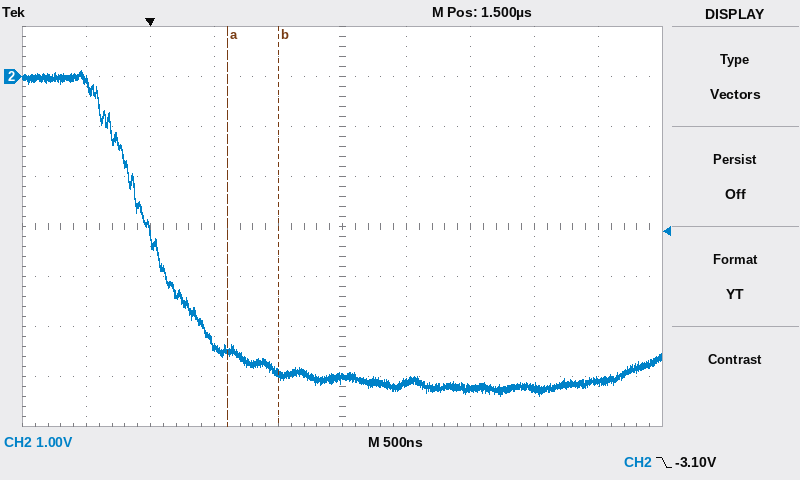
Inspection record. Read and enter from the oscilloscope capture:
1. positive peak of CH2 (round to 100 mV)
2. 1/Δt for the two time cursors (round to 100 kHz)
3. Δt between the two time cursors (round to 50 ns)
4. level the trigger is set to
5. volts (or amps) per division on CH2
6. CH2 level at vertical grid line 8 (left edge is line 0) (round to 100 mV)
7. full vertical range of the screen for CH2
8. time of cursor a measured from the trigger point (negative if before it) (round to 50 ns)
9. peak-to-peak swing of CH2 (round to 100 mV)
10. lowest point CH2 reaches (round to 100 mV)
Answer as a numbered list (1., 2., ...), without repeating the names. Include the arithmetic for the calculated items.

1. 100 mV
2. 1 / 400 ns ≈ 2.5 MHz
3. 400 ns
4. -3.10 V
5. 1 V
6. -6.2 V
7. 8 V
8. +600 ns
9. 100 mV − (-6.4 V) = 6.5 V
10. -6.4 V
